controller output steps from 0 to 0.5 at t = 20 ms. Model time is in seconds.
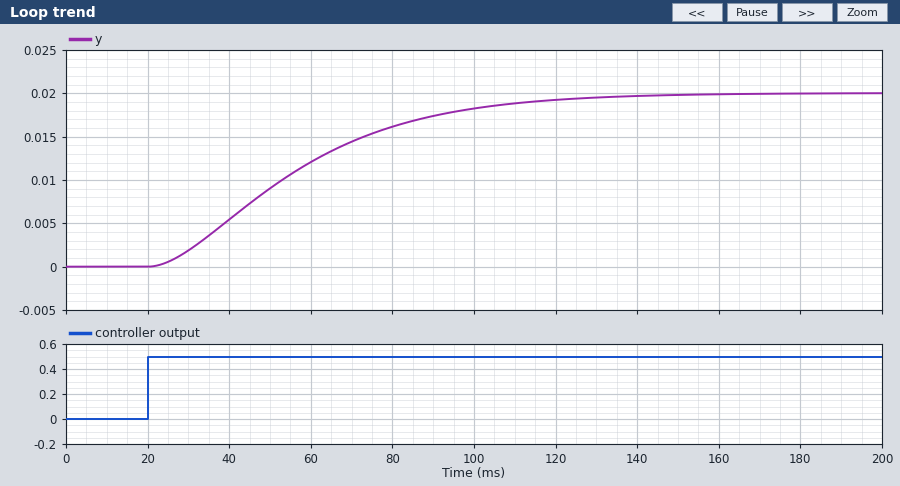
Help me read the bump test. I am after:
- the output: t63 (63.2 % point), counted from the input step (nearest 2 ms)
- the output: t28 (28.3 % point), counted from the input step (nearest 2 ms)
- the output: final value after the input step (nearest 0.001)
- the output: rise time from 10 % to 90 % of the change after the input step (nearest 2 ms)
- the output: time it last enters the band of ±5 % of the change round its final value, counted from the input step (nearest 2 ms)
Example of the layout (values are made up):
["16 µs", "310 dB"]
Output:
["42 ms", "20 ms", "0.020", "66 ms", "94 ms"]
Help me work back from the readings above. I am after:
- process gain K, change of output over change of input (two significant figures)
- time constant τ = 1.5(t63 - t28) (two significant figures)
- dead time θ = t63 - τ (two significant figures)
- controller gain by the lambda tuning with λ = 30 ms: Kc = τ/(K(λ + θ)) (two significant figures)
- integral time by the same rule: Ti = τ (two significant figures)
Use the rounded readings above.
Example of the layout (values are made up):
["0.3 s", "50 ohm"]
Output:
["0.040", "33 ms", "9.0 ms", "21", "33 ms"]
